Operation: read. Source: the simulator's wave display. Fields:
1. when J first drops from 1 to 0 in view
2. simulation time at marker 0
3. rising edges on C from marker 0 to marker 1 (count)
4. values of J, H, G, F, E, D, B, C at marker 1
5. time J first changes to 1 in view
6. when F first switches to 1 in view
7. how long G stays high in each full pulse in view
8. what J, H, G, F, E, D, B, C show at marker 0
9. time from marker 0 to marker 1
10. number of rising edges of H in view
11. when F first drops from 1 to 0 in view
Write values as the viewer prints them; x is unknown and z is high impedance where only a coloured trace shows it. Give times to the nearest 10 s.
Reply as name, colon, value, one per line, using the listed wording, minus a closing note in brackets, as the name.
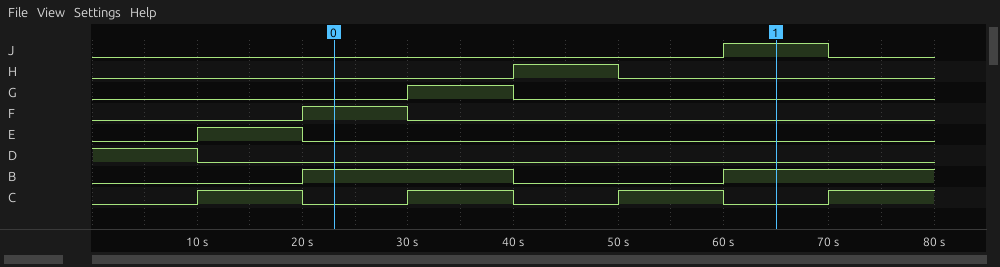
when J first drops from 1 to 0 in view: 70 s
simulation time at marker 0: 20 s
rising edges on C from marker 0 to marker 1: 2
values of J, H, G, F, E, D, B, C at marker 1: J=1, H=0, G=0, F=0, E=0, D=0, B=1, C=0
time J first changes to 1 in view: 60 s
when F first switches to 1 in view: 20 s
how long G stays high in each full pulse in view: 10 s
what J, H, G, F, E, D, B, C show at marker 0: J=0, H=0, G=0, F=1, E=0, D=0, B=1, C=0
time from marker 0 to marker 1: 40 s
number of rising edges of H in view: 1
when F first drops from 1 to 0 in view: 30 s
